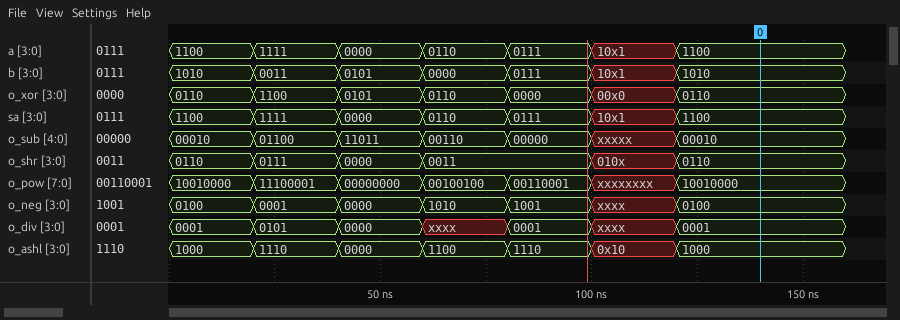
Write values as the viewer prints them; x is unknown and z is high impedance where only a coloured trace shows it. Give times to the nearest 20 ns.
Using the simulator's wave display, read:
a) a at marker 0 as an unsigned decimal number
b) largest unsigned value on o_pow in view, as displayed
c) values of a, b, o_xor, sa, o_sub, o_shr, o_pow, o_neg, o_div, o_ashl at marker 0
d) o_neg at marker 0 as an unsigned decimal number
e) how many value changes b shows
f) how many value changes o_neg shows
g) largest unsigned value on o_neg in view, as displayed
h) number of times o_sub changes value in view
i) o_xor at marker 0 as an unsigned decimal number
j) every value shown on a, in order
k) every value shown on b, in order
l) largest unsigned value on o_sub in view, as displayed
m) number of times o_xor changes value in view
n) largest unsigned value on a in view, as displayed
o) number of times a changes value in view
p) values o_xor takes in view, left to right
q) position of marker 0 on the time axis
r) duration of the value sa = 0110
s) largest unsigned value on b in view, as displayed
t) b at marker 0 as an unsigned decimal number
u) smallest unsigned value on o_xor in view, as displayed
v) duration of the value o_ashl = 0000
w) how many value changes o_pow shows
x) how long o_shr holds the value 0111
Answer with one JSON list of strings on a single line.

["12", "11100001", "a=1100, b=1010, o_xor=0110, sa=1100, o_sub=00010, o_shr=0110, o_pow=10010000, o_neg=0100, o_div=0001, o_ashl=1000", "4", "6", "6", "1010", "6", "6", "1100, 1111, 0000, 0110, 0111, 10x1, 1100", "1010, 0011, 0101, 0000, 0111, 10x1, 1010", "11011", "6", "1111", "6", "0110, 1100, 0101, 0110, 0000, 00x0, 0110", "140 ns", "20 ns", "1010", "10", "0000", "20 ns", "6", "20 ns"]
